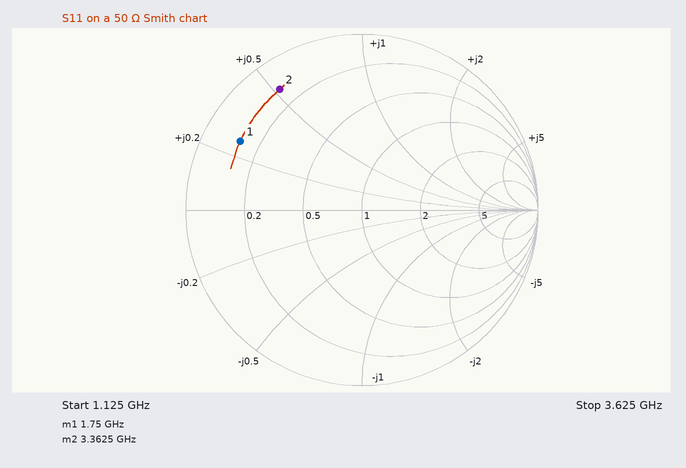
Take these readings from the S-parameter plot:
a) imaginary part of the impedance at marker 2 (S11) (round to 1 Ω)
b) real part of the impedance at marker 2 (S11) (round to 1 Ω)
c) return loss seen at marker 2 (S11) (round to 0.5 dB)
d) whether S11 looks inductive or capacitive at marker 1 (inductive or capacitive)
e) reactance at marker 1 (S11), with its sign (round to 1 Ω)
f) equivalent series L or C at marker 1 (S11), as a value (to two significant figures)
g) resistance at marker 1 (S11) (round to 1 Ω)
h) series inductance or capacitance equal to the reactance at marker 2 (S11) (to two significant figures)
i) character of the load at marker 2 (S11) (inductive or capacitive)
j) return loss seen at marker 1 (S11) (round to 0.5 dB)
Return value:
+26 Ω
6 Ω
1.5 dB
inductive
+13 Ω
1.2 nH
6 Ω
1.2 nH
inductive
2.0 dB
